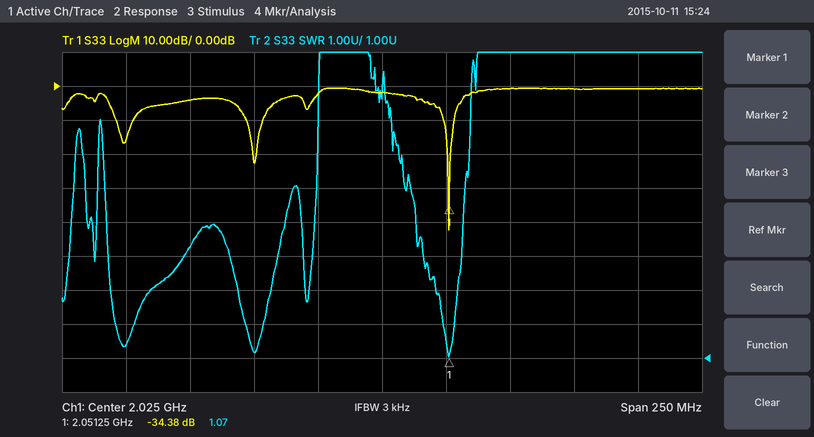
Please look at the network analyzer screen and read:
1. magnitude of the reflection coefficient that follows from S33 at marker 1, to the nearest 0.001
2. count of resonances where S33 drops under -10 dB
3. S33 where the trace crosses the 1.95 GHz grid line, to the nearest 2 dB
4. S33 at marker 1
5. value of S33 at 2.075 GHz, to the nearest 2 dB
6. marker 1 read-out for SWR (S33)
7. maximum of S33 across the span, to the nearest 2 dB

0.019
3
-4 dB
-34.38 dB
0 dB
1.07
0 dB
